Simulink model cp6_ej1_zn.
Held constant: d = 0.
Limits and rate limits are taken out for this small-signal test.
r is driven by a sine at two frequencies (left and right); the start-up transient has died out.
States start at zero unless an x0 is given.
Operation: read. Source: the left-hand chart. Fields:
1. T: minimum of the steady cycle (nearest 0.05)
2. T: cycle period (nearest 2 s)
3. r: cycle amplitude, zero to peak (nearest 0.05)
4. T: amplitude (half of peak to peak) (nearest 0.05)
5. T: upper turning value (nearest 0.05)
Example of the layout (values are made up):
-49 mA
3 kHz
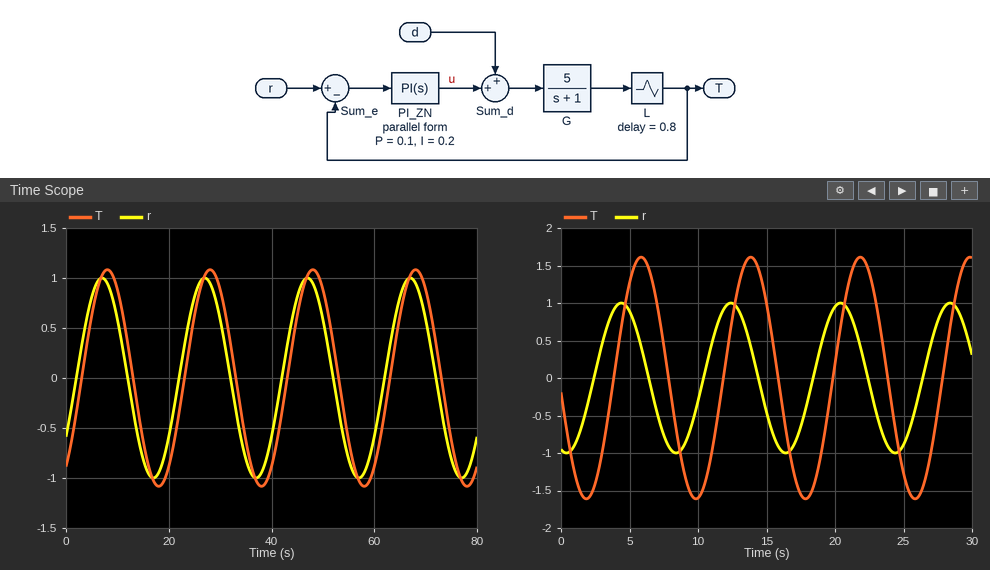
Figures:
-1.10
20 s
1.00
1.10
1.10
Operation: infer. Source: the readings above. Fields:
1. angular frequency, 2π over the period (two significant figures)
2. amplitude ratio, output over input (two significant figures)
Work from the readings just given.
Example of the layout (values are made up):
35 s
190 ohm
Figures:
0.31 rad/s
1.1
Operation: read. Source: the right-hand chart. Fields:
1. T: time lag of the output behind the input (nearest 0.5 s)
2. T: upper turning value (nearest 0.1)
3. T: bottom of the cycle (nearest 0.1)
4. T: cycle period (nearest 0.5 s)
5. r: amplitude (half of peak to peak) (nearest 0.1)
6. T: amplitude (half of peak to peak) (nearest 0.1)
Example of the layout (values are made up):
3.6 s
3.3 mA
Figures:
1.5 s
1.6
-1.6
8.0 s
1.0
1.6
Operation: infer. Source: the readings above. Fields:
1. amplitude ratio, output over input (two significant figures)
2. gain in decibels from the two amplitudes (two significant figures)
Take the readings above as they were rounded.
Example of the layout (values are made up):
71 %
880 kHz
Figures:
1.6
4.1 dB
